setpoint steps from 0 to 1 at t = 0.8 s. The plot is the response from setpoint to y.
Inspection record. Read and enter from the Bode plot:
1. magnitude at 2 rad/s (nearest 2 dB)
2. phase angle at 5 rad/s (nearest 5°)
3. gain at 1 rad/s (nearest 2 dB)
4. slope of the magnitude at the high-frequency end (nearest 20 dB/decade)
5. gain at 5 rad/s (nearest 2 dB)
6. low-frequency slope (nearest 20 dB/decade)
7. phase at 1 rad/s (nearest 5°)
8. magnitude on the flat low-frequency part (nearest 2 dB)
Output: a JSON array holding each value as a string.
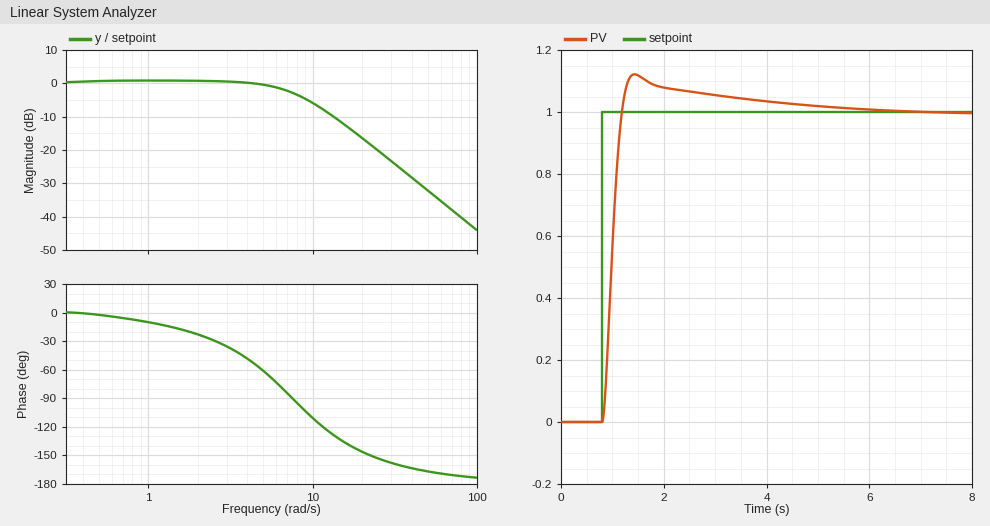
["0 dB", "-60°", "0 dB", "-40 dB/decade", "0 dB", "0 dB/decade", "-10°", "0 dB"]
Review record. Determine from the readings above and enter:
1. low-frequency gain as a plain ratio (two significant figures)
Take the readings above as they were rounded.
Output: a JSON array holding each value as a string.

["1.0"]
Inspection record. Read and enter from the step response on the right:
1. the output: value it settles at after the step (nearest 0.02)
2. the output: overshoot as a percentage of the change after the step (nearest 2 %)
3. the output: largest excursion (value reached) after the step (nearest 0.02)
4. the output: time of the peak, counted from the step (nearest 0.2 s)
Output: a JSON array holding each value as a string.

["1.00", "12 %", "1.12", "0.6 s"]
